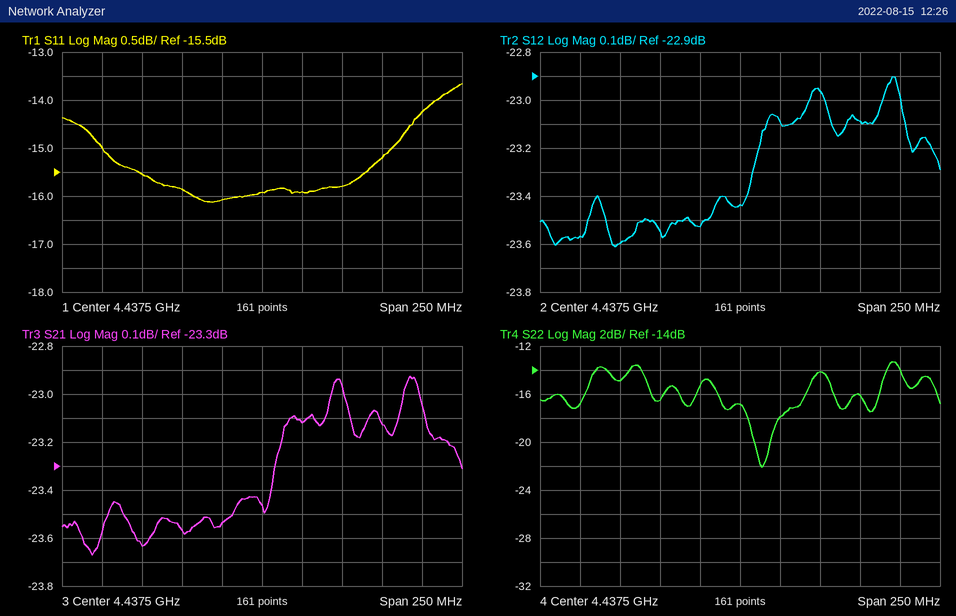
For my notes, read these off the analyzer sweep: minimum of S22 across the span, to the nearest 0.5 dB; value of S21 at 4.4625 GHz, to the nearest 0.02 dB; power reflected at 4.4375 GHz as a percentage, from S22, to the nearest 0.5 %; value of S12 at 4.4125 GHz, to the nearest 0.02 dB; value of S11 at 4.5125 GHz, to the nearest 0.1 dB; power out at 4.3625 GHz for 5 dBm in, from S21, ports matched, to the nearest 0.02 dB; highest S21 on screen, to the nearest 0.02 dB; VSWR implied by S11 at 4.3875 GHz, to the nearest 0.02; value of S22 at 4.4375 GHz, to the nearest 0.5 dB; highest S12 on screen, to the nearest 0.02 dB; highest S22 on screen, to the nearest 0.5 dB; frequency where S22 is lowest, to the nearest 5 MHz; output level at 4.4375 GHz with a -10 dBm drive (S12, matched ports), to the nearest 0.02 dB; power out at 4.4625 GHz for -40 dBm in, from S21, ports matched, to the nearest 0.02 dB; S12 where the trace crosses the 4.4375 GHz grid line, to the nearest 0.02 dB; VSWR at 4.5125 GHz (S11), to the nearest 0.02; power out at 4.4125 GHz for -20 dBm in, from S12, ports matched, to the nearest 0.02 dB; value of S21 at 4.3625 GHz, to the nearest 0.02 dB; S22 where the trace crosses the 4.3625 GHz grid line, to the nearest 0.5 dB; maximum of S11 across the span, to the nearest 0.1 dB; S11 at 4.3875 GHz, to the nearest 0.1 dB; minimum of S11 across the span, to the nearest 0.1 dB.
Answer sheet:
-22.0 dB
-23.12 dB
2.0 %
-23.52 dB
-15.2 dB
-18.64 dBm
-22.92 dB
1.38
-17.0 dB
-22.90 dB
-13.5 dB
4.450 GHz
-33.44 dBm
-63.12 dBm
-23.44 dB
1.42
-43.52 dBm
-23.64 dB
-15.0 dB
-13.7 dB
-15.9 dB
-16.1 dB
